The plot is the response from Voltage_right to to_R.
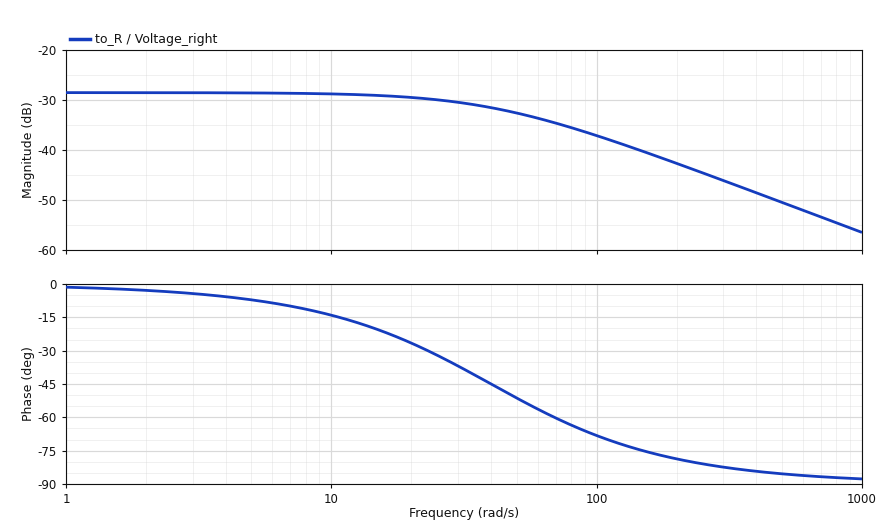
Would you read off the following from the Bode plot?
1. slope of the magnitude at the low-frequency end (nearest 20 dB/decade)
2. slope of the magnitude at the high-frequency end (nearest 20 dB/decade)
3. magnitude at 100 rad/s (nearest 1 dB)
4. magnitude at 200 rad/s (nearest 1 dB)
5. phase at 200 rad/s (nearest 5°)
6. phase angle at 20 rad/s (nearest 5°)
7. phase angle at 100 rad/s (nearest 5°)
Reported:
0 dB/decade
-20 dB/decade
-37 dB
-43 dB
-80°
-25°
-70°
